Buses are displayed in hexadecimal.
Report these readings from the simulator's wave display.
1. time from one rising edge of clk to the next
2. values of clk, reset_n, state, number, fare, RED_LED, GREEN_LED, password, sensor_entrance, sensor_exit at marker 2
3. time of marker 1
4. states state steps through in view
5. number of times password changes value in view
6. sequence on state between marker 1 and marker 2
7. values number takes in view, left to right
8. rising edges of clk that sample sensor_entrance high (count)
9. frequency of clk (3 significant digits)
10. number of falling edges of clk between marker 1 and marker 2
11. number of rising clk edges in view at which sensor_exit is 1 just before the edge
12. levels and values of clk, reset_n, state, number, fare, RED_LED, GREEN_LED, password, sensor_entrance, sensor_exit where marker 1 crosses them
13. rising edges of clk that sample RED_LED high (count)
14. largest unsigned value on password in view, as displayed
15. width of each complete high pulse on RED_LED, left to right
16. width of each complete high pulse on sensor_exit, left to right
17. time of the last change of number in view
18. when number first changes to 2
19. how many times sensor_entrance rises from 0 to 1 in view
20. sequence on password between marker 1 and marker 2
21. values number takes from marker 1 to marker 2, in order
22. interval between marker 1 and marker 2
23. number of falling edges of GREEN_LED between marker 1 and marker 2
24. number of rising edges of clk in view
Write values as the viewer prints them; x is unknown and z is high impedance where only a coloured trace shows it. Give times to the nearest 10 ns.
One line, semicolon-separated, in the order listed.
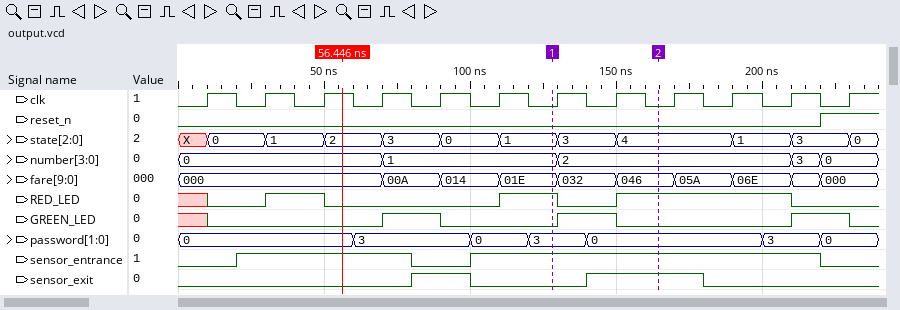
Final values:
20 ns; clk=0, reset_n=0, state=4, number=2, fare=046, RED_LED=1, GREEN_LED=0, password=0, sensor_entrance=1, sensor_exit=1; 130 ns; X, 0, 1, 2, 3, 0, 1, 3, 4, 1, 3, 0; 6; 1, 3, 4; 0, 1, 2, 3, 0; 9; 50.0 MHz; 2; 3; clk=0, reset_n=0, state=1, number=1, fare=01E, RED_LED=1, GREEN_LED=0, password=3, sensor_entrance=1, sensor_exit=0; 5; 3; 20 ns, 20 ns, 60 ns; 20 ns, 40 ns; 220 ns; 130 ns; 2; 3, 0; 1, 2; 40 ns; 1; 12
